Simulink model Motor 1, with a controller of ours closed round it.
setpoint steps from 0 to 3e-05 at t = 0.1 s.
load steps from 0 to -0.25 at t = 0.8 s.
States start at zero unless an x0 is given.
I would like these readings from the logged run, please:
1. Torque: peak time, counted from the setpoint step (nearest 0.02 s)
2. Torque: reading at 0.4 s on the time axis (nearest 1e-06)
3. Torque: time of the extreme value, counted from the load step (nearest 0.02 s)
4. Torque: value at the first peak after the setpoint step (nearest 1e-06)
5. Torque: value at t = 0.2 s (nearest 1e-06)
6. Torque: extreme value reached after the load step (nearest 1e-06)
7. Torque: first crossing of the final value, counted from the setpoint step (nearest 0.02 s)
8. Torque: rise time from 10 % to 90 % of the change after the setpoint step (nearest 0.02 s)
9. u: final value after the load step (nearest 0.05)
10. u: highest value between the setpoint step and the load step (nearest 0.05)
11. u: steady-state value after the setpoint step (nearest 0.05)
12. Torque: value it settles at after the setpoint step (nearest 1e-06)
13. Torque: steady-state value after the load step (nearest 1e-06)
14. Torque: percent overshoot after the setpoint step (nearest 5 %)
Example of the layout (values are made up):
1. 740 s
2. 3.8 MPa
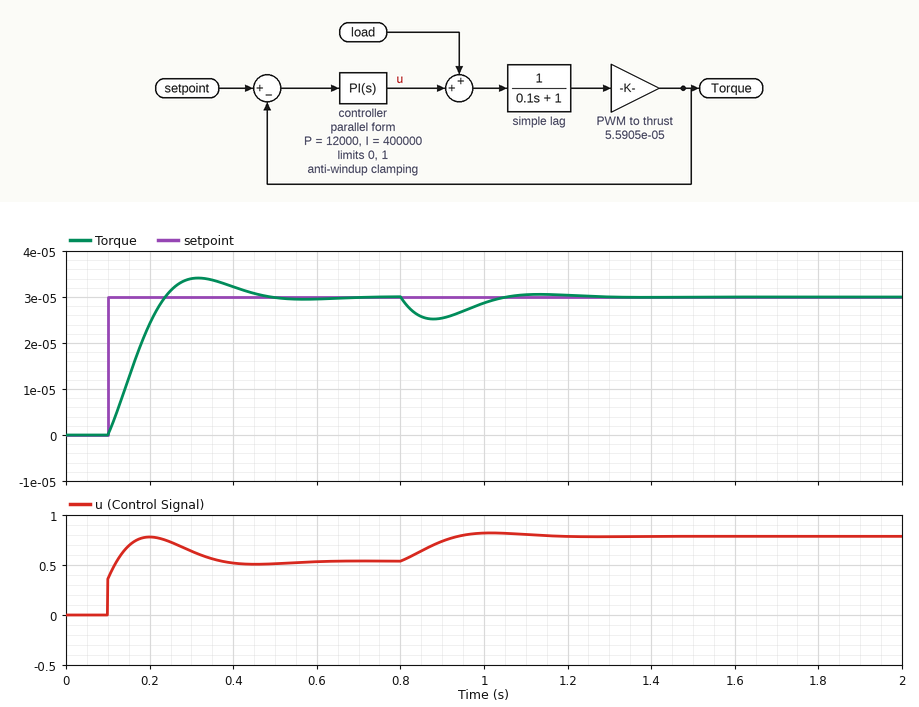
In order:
1. 0.22 s
2. 0.000032
3. 0.08 s
4. 0.000034
5. 0.000024
6. 0.000025
7. 0.14 s
8. 0.10 s
9. 0.80
10. 0.80
11. 0.55
12. 0.000030
13. 0.000030
14. 15 %
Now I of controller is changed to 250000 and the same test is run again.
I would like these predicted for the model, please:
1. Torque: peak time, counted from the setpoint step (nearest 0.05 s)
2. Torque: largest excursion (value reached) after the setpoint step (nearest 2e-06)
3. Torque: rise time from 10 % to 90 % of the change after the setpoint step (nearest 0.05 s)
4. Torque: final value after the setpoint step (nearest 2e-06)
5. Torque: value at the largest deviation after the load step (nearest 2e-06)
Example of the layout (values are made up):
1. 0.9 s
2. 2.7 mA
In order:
1. 0.30 s
2. 0.000032
3. 0.15 s
4. 0.000030
5. 0.000024
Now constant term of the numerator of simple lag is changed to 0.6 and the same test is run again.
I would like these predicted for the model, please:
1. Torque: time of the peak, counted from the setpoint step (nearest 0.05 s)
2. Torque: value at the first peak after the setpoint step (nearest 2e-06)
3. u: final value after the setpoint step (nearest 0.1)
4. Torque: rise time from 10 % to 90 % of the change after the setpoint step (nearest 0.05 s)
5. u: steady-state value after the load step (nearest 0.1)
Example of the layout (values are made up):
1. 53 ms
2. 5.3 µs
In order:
1. 0.35 s
2. 0.000032
3. 0.9
4. 0.15 s
5. 1.0
